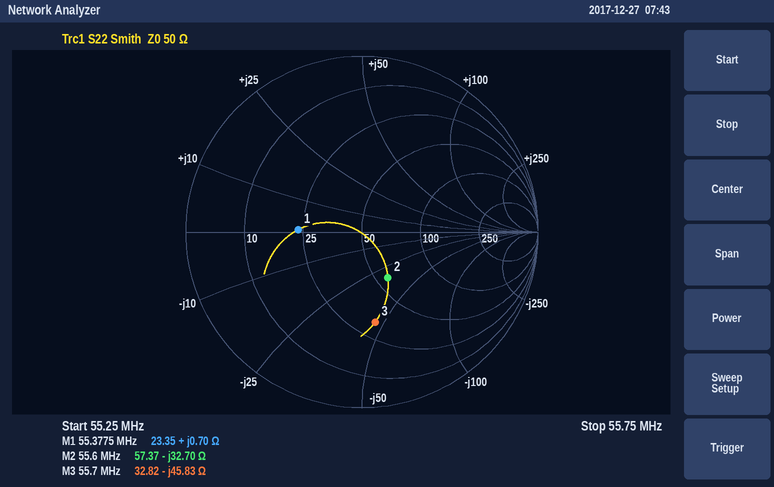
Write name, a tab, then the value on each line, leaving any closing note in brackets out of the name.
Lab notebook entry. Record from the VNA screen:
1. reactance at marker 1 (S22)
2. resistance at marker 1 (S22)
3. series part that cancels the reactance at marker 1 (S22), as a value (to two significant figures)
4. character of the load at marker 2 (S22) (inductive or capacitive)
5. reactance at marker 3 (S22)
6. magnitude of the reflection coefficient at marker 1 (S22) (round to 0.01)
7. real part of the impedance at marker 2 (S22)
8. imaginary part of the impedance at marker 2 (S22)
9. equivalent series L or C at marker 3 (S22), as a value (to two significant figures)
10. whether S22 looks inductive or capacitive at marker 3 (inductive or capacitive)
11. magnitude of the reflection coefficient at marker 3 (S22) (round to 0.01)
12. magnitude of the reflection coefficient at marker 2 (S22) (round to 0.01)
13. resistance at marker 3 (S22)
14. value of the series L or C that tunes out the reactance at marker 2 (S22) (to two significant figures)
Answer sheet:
reactance at marker 1	+0.70 Ω
resistance at marker 1	23.35 Ω
series part that cancels the reactance at marker 1 (S22), as a value	4.1 nF
character of the load at marker 2 (S22)	capacitive
reactance at marker 3	-45.83 Ω
magnitude of the reflection coefficient at marker 1 (S22)	0.36
real part of the impedance at marker 2	57.37 Ω
imaginary part of the impedance at marker 2	-32.70 Ω
equivalent series L or C at marker 3 (S22), as a value	62 pF
whether S22 looks inductive or capacitive at marker 3	capacitive
magnitude of the reflection coefficient at marker 3 (S22)	0.52
magnitude of the reflection coefficient at marker 2 (S22)	0.30
resistance at marker 3	32.82 Ω
value of the series L or C that tunes out the reactance at marker 2 (S22)	94 nH
